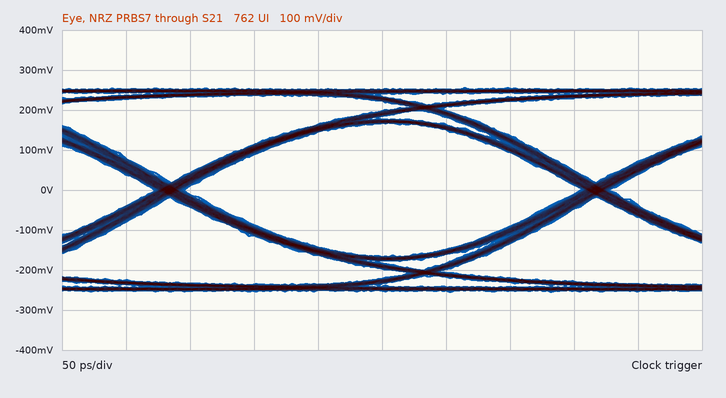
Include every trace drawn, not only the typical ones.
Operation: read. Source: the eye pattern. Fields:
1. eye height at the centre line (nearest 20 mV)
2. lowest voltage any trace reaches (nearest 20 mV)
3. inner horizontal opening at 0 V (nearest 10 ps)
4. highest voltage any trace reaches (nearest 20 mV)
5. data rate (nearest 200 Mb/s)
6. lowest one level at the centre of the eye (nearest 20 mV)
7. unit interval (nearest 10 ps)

340 mV
-260 mV
310 ps
260 mV
3.0 Gb/s
160 mV
330 ps
